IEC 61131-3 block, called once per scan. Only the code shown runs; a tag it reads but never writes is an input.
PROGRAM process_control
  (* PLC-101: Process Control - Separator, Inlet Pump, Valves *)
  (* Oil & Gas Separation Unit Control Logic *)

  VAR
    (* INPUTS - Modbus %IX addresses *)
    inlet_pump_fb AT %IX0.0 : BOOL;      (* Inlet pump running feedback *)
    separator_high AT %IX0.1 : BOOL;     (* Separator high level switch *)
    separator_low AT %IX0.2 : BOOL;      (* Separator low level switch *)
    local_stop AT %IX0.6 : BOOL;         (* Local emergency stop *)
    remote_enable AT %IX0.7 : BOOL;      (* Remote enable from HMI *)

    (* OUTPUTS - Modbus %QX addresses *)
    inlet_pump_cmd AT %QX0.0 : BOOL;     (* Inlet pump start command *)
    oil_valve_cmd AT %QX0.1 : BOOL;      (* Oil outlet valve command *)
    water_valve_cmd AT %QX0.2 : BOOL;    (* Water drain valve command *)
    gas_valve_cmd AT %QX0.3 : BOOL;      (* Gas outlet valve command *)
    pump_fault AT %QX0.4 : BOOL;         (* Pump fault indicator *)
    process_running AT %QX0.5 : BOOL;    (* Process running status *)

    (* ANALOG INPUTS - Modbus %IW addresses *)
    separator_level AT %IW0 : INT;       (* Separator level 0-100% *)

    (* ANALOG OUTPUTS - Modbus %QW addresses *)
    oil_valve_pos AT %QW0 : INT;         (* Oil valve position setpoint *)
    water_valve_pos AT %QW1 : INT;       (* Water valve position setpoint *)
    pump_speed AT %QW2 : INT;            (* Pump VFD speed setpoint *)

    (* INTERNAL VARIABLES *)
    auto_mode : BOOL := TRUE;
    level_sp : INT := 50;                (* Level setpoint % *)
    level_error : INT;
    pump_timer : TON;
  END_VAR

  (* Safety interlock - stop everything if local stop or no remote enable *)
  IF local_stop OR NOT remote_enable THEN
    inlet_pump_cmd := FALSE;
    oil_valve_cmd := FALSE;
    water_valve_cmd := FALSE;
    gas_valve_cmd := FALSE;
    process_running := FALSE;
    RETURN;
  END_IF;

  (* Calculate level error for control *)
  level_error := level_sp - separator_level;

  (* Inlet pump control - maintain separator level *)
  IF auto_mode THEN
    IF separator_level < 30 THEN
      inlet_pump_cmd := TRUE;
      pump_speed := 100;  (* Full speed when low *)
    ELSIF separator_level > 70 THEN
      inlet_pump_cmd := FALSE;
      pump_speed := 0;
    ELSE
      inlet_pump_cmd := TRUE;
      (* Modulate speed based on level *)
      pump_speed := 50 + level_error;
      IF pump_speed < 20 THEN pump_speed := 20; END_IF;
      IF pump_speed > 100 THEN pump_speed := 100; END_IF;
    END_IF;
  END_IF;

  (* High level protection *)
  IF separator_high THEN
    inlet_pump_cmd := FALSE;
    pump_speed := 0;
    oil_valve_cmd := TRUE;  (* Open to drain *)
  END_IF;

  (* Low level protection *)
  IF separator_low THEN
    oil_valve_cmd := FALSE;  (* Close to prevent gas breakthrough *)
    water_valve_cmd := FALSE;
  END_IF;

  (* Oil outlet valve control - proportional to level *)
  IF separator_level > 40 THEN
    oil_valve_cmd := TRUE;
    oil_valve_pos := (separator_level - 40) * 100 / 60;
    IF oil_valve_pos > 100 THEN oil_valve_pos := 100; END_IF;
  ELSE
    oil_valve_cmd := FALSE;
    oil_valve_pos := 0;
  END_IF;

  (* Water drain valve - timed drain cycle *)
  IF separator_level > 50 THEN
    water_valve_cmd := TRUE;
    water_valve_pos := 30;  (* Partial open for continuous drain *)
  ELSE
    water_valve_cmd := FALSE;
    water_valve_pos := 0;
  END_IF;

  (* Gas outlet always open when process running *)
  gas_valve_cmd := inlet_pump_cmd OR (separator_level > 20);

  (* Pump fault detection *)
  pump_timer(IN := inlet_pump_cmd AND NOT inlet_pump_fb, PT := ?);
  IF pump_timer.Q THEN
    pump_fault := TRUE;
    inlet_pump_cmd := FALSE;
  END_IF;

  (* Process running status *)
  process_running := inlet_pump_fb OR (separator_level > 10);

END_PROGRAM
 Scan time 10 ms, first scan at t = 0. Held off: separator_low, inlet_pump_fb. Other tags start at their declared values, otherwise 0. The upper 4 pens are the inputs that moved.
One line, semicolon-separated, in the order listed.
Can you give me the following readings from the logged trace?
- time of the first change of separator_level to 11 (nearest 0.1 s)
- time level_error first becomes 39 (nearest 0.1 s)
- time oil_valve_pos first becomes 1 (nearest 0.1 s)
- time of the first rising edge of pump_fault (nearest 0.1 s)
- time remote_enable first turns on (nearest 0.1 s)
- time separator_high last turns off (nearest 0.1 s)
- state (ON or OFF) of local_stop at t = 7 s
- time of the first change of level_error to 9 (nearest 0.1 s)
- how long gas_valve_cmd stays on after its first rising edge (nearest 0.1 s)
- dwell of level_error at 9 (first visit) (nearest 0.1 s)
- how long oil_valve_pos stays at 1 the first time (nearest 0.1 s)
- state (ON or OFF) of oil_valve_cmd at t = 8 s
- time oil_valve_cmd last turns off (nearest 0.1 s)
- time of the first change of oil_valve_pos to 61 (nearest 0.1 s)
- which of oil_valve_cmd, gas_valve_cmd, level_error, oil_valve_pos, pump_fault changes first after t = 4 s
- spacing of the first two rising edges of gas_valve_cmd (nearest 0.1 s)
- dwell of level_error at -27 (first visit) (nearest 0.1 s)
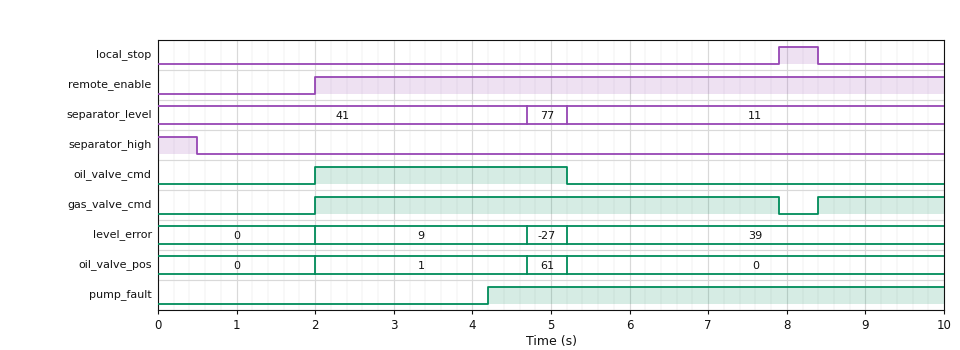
5.2 s; 5.2 s; 2.0 s; 4.2 s; 2.0 s; 0.5 s; OFF; 2.0 s; 5.9 s; 2.7 s; 2.7 s; OFF; 5.2 s; 4.7 s; pump_fault; 6.4 s; 0.5 s
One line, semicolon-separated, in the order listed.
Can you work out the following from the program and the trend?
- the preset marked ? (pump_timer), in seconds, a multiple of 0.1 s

2.2 s
